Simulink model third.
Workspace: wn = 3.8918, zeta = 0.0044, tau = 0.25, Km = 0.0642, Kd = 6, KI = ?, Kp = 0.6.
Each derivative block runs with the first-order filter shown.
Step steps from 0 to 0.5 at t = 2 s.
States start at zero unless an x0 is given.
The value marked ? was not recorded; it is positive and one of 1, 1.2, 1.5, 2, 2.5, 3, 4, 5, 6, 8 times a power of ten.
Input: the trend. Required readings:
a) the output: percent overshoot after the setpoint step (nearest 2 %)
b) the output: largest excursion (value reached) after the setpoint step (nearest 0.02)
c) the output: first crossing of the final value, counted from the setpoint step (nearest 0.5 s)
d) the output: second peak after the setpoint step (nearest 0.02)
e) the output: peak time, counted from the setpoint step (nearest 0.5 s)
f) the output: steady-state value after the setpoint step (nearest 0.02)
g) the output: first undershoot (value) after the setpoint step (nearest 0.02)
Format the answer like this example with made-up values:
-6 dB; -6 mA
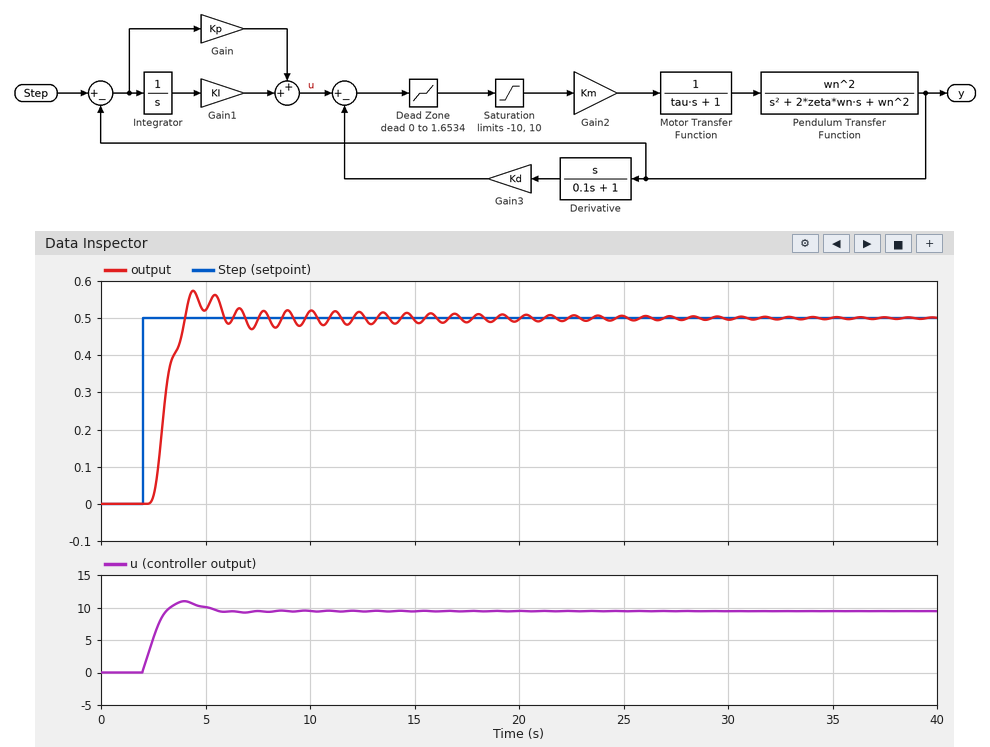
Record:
14 %; 0.58; 2.0 s; 0.56; 2.5 s; 0.50; 0.52
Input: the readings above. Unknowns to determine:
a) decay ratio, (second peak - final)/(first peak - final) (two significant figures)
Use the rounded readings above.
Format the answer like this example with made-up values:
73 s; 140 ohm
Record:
0.75
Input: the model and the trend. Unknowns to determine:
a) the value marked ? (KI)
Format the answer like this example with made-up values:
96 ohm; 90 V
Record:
20
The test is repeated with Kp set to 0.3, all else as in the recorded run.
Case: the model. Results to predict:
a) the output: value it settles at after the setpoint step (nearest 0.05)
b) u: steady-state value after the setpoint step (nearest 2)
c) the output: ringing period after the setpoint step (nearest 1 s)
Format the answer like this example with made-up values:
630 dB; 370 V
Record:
0.50; 10; 3 s
